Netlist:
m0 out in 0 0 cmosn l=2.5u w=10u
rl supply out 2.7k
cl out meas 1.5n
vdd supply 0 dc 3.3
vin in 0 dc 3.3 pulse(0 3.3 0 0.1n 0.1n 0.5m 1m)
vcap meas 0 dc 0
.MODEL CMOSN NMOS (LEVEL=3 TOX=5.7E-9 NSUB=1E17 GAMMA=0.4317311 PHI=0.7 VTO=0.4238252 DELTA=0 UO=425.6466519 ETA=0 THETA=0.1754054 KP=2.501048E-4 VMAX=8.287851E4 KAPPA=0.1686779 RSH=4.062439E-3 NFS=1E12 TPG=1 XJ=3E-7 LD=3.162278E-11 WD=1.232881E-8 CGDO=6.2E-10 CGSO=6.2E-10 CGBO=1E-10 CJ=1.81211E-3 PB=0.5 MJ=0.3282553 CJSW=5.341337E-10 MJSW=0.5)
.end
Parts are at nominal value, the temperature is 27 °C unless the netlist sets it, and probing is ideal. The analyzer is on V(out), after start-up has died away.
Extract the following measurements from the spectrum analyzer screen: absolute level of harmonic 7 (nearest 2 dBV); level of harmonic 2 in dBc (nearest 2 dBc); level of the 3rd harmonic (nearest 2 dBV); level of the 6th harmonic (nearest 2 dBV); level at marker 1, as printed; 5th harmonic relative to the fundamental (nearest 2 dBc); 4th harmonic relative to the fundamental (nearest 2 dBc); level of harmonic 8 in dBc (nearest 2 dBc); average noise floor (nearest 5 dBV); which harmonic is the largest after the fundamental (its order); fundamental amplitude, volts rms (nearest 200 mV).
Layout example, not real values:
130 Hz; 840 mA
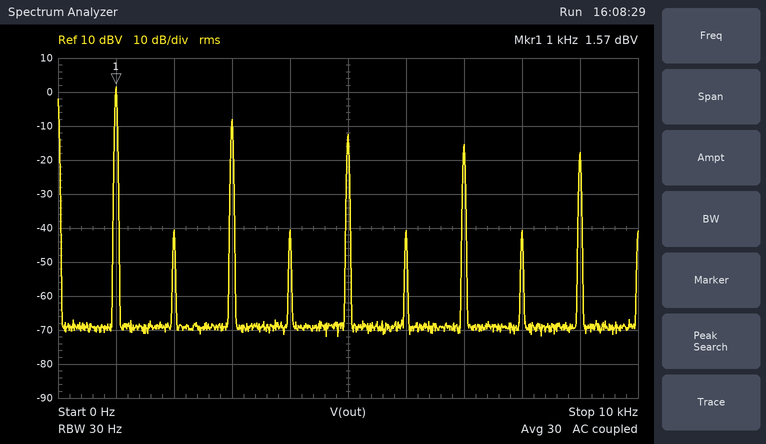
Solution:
-16 dBV; -42 dBc; -8 dBV; -40 dBV; 1.57 dBV; -14 dBc; -42 dBc; -42 dBc; -70 dBV; 3; 1.2 V
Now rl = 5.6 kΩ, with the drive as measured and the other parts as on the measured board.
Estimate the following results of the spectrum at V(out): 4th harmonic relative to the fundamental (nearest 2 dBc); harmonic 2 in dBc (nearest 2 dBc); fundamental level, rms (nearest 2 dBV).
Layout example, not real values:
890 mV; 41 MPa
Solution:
-34 dBc; -34 dBc; 2 dBV
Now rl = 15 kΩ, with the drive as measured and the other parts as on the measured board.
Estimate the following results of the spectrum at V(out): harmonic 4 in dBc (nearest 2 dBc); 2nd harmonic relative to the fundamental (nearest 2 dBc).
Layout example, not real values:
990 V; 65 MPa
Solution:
-24 dBc; -24 dBc
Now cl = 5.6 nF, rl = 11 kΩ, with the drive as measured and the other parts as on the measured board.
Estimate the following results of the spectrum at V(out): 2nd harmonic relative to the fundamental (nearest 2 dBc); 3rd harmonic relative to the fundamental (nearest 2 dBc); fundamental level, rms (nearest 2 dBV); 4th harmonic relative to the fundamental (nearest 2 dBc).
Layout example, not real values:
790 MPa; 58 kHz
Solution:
-16 dBc; -12 dBc; 2 dBV; -20 dBc
